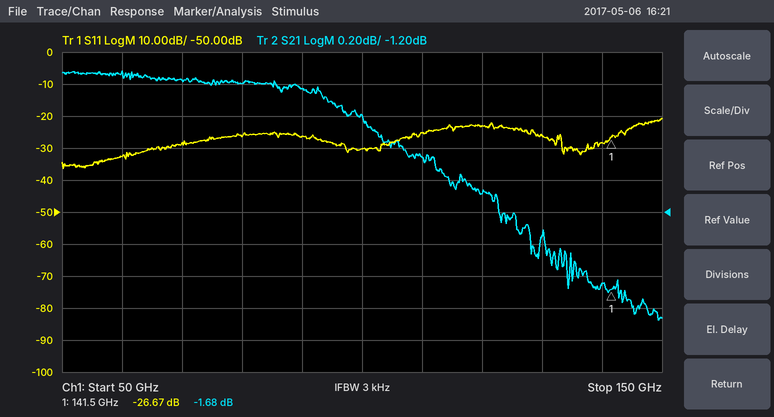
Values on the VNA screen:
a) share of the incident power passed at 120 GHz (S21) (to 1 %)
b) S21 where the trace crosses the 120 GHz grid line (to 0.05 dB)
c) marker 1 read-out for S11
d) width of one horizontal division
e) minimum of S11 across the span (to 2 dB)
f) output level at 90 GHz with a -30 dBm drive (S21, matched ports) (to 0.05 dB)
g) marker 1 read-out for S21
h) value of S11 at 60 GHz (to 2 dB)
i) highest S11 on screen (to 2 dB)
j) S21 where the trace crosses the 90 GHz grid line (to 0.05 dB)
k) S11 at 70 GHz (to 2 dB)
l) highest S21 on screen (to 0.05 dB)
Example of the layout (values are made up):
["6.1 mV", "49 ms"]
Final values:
["78 %", "-1.10 dB", "-26.67 dB", "10 GHz", "-36 dB", "-30.45 dBm", "-1.68 dB", "-32 dB", "-20 dB", "-0.45 dB", "-28 dB", "-0.30 dB"]
